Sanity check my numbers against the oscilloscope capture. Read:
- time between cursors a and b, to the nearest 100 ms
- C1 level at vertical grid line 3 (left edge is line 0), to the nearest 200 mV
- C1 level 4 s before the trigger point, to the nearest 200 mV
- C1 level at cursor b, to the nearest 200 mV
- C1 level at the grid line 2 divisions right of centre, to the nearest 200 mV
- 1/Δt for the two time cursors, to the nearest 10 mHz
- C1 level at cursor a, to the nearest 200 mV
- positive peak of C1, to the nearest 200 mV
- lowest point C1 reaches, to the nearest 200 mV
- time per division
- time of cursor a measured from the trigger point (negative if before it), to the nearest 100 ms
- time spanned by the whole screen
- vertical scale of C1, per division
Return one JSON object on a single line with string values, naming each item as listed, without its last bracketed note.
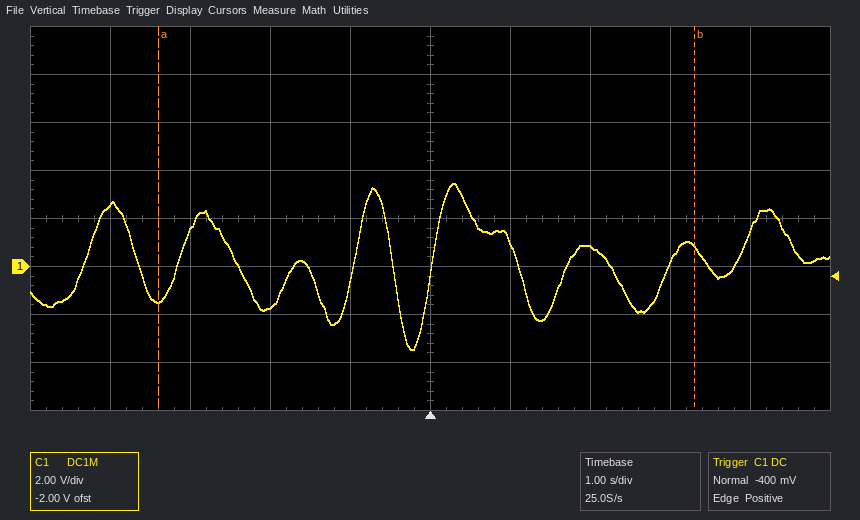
{"time between cursors a and b, to the nearest 100 ms": "6.7 s", "C1 level at vertical grid line 3 (left edge is line 0), to the nearest 200 mV": "-1.6 V", "C1 level 4 s before the trigger point, to the nearest 200 mV": "2.6 V", "C1 level at cursor b, to the nearest 200 mV": "800 mV", "C1 level at the grid line 2 divisions right of centre, to the nearest 200 mV": "800 mV", "1/Δt for the two time cursors, to the nearest 10 mHz": "150 mHz", "C1 level at cursor a, to the nearest 200 mV": "-1.4 V", "positive peak of C1, to the nearest 200 mV": "3.4 V", "lowest point C1 reaches, to the nearest 200 mV": "-3.4 V", "time per division": "1 s", "time of cursor a measured from the trigger point (negative if before it), to the nearest 100 ms": "-3.4 s", "time spanned by the whole screen": "10 s", "vertical scale of C1, per division": "2 V"}
